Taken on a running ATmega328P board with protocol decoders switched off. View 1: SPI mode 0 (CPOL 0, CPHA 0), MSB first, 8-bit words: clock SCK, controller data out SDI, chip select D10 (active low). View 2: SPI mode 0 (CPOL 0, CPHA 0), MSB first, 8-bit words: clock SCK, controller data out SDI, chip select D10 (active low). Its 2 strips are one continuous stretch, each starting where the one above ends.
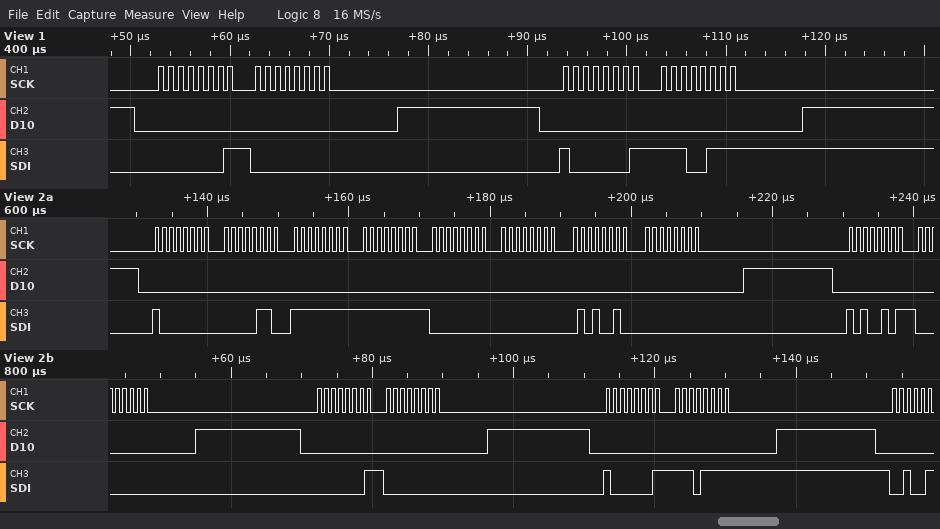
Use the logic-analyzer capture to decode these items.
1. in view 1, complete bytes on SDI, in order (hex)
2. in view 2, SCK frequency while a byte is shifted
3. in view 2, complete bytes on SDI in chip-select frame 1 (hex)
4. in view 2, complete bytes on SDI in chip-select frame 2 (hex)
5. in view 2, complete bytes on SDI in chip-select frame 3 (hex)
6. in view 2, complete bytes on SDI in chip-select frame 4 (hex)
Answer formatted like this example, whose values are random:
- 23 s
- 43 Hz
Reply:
- 01 00 81 E7
- 1 MHz
- 80 06 FF FF 00 00 52 00
- A5 00
- 01 00
- 81 EF
